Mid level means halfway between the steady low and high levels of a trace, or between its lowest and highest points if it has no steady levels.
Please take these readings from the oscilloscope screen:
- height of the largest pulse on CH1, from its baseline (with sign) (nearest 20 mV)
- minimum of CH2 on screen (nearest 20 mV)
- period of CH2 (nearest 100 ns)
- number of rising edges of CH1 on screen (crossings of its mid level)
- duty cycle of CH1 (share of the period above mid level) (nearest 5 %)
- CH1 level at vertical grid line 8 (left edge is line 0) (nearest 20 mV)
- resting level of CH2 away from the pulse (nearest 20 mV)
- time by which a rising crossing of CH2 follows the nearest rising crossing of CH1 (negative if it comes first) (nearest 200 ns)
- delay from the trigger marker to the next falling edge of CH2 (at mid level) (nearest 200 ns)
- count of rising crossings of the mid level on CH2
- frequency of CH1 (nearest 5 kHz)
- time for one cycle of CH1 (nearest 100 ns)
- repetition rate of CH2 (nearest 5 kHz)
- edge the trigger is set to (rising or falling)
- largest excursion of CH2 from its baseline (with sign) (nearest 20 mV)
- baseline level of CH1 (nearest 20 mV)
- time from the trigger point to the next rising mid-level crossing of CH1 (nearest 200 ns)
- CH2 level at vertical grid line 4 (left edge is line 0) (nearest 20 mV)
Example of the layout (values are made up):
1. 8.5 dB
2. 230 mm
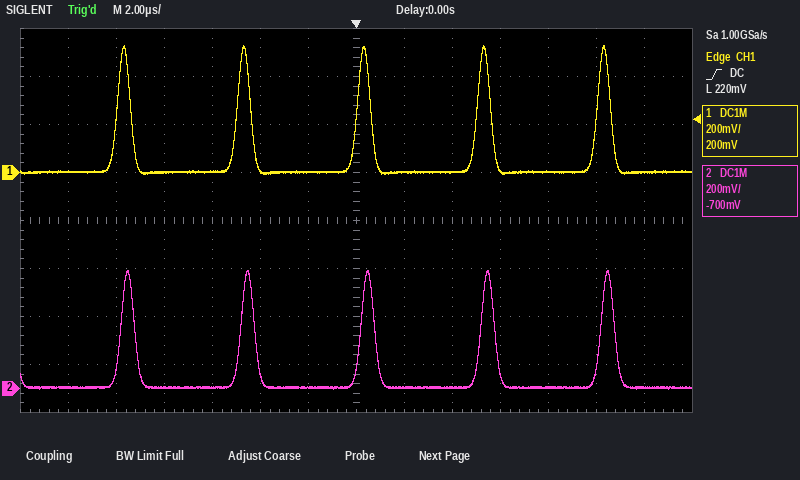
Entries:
1. +520 mV
2. 0 mV
3. 5.0 µs
4. 5
5. 10 %
6. 0 mV
7. 0 mV
8. +200 ns
9. 800 ns
10. 5
11. 200 kHz
12. 5.0 µs
13. 200 kHz
14. rising
15. +480 mV
16. 0 mV
17. 5.0 µs
18. 0 mV
